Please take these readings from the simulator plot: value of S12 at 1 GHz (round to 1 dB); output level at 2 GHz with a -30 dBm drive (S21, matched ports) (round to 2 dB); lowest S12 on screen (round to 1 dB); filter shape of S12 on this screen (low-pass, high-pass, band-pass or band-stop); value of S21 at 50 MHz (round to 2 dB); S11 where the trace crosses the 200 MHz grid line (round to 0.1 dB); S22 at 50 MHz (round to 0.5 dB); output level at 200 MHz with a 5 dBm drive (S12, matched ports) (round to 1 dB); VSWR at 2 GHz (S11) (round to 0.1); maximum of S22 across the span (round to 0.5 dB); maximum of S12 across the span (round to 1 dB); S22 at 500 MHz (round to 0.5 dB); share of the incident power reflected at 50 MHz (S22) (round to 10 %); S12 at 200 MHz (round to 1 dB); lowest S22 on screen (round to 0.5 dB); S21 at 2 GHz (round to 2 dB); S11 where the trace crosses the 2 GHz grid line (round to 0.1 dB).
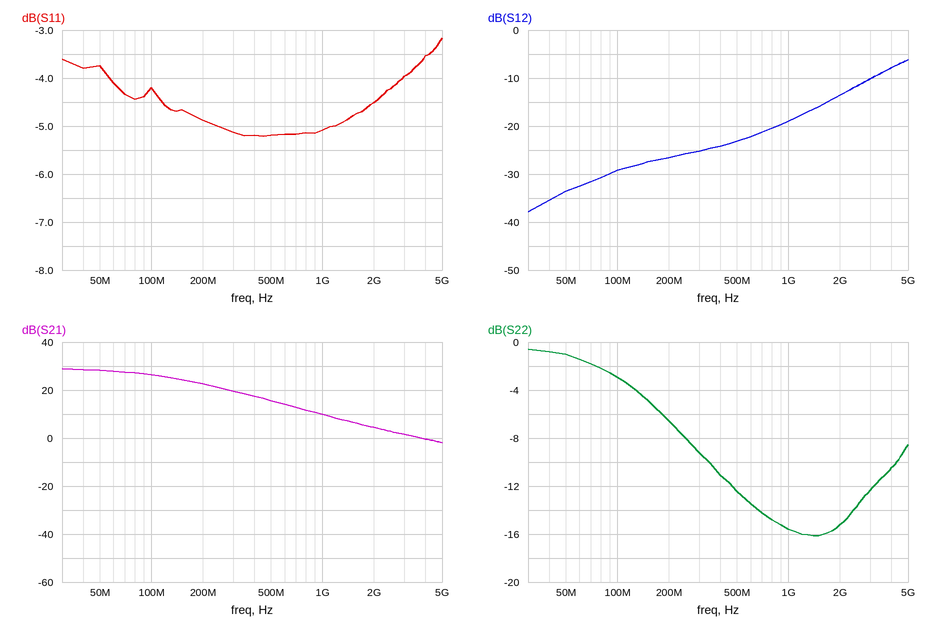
-19 dB
-26 dBm
-38 dB
high-pass
28 dB
-4.9 dB
-1.0 dB
-22 dBm
3.9
-0.5 dB
-6 dB
-12.5 dB
80 %
-27 dB
-16.0 dB
4 dB
-4.5 dB
